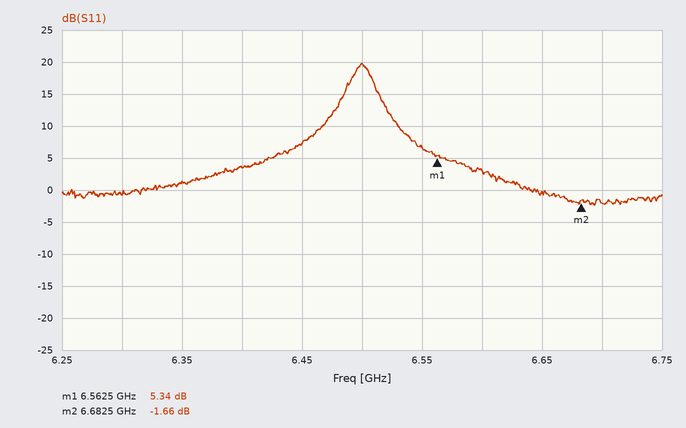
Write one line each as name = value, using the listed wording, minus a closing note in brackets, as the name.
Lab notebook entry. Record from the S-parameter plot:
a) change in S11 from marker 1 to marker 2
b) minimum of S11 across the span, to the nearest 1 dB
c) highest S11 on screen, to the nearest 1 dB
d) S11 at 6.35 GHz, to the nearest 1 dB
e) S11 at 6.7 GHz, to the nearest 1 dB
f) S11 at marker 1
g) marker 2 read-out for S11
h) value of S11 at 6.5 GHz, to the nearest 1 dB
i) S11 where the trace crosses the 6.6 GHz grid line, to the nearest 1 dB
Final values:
change in S11 from marker 1 to marker 2 = -7.00 dB
minimum of S11 across the span, to the nearest 1 dB = -2 dB
highest S11 on screen, to the nearest 1 dB = 20 dB
S11 at 6.35 GHz, to the nearest 1 dB = 1 dB
S11 at 6.7 GHz, to the nearest 1 dB = -2 dB
S11 at marker 1 = 5.34 dB
marker 2 read-out for S11 = -1.66 dB
value of S11 at 6.5 GHz, to the nearest 1 dB = 20 dB
S11 where the trace crosses the 6.6 GHz grid line, to the nearest 1 dB = 3 dB
